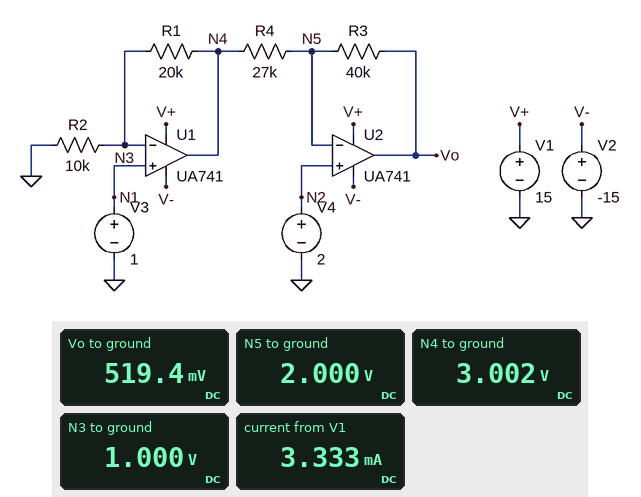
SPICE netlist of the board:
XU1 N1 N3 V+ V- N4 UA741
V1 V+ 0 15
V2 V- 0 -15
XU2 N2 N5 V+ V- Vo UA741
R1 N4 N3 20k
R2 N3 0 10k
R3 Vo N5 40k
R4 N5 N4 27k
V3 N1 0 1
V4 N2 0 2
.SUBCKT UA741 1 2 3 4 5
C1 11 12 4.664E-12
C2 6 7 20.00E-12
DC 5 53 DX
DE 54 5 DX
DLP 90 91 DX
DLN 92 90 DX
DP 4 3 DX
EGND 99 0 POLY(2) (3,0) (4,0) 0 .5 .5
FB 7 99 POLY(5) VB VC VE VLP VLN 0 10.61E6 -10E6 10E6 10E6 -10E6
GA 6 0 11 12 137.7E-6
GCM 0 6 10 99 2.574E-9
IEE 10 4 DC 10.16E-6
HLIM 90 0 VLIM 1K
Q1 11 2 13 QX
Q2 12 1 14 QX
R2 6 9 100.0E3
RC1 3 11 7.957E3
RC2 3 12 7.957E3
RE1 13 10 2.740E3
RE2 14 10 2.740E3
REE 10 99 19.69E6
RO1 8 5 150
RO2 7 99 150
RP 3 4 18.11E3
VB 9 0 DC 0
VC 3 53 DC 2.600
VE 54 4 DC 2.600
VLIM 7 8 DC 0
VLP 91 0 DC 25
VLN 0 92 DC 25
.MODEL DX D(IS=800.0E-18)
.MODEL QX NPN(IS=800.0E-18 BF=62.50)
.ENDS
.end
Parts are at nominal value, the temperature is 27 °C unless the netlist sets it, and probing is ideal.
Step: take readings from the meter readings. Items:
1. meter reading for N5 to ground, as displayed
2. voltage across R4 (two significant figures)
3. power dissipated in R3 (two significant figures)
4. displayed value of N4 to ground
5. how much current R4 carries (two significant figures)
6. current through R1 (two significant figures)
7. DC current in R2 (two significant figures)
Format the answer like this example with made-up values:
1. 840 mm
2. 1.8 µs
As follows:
1. 2.000 V
2. 1.0 V
3. 55 µW
4. 3.002 V
5. 37 µA
6. 100 µA
7. 100 µA
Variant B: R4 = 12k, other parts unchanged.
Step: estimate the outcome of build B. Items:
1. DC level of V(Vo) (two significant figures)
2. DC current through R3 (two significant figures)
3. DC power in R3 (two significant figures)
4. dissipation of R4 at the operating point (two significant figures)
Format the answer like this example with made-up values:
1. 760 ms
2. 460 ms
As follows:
1. -1.3 V
2. 83 µA
3. 280 µW
4. 84 µW
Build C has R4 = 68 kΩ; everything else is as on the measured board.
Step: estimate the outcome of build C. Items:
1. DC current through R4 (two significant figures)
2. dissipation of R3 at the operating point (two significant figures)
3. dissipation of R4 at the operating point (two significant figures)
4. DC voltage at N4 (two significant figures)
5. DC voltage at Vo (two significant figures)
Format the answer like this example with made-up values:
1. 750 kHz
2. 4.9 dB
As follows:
1. 15 µA
2. 8.6 µW
3. 15 µW
4. 3.0 V
5. 1.4 V
